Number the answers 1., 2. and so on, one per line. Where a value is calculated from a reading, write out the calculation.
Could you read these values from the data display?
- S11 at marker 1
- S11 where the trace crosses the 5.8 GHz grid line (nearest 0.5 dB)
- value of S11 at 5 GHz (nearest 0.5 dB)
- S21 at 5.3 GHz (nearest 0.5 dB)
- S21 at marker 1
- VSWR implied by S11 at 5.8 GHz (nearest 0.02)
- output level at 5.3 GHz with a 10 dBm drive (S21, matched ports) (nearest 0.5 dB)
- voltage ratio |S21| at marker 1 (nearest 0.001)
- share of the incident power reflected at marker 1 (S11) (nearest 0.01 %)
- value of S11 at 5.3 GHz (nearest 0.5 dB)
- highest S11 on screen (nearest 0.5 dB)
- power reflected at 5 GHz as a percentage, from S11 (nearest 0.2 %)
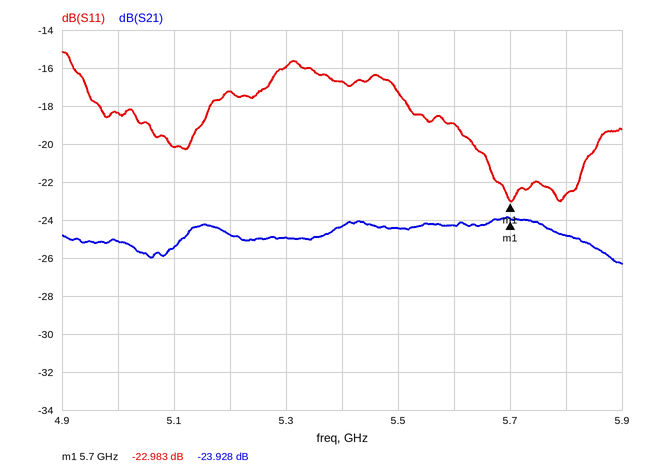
1. -22.983 dB
2. -22.5 dB
3. -18.5 dB
4. -25.0 dB
5. -23.928 dB
6. |Γ| = 10^(-22.5/20) = 0.0750; VSWR = (1 + 0.0750)/(1 − 0.0750) ≈ 1.16
7. 10 dBm + (-25.0 dB) = -15.0 dBm
8. 10^(-23.928/20) ≈ 0.064
9. 10^(-22.983/10) ≈ 0.50 %
10. -16.0 dB
11. -15.0 dB
12. 10^(-18.5/10) ≈ 1.4 %
